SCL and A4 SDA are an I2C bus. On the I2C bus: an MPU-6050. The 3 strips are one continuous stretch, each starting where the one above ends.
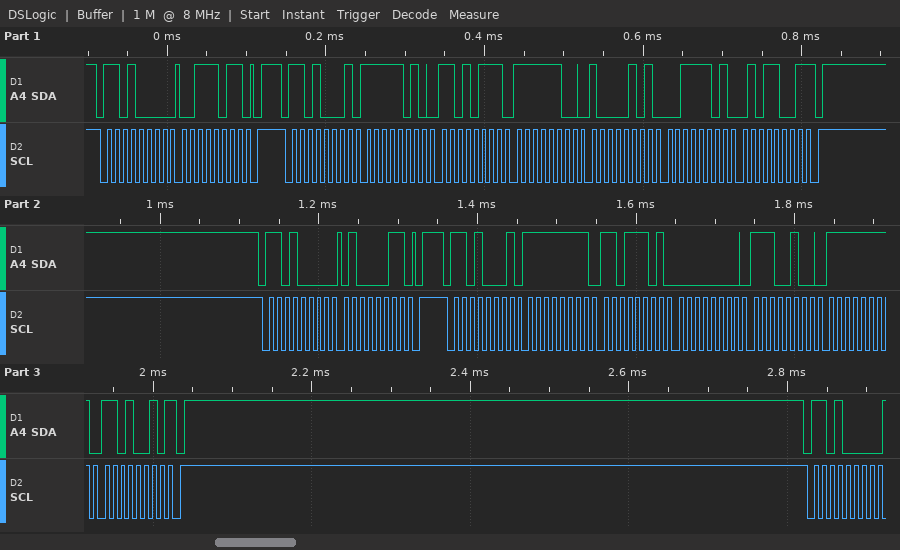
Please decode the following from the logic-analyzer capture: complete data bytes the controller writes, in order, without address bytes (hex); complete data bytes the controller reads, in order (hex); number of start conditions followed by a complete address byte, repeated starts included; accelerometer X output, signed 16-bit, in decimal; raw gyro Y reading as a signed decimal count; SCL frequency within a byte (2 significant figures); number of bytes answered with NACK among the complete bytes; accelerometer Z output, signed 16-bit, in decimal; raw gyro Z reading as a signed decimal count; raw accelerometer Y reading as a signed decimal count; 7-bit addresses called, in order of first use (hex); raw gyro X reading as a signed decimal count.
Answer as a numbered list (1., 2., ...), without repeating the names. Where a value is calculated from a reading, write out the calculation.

1. 3B 43
2. FA D7 FC 85 3D 59 FF DD 00 E4 FF D2
3. 5
4. 0xFAD7 = -1321
5. 0x00E4 = 228
6. 100 kHz
7. 2
8. 0x3D59 = 15705
9. 0xFFD2 = -46
10. 0xFC85 = -891
11. 0x68
12. 0xFFDD = -35
